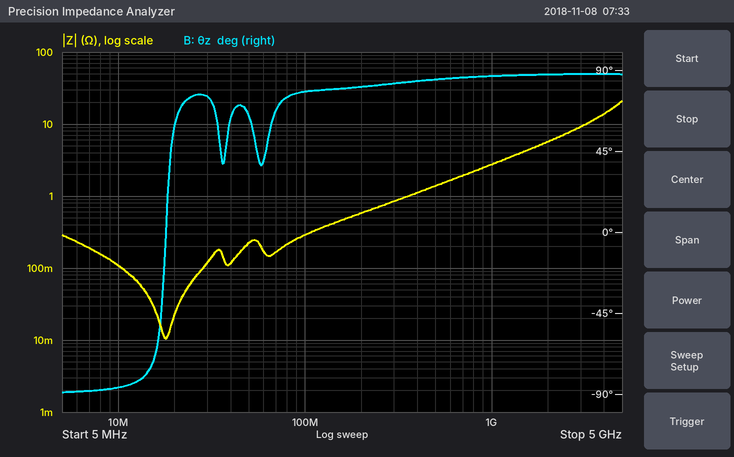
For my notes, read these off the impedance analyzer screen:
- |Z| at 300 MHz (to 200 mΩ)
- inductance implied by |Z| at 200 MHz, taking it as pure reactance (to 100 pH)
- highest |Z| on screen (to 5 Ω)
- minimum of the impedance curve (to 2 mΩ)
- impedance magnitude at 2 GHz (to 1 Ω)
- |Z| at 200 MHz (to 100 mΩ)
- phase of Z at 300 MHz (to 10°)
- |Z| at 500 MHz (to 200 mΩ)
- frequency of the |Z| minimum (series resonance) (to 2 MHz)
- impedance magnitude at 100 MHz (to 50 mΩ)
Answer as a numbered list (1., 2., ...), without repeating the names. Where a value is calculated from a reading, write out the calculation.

1. 800 mΩ
2. L = 600 mΩ/(2π × 200 MHz) ≈ 477 pH, so 500 pH to the nearest 100 pH
3. 20 Ω
4. 10 mΩ
5. 6 Ω
6. 600 mΩ
7. 80°
8. 1.4 Ω
9. 18 MHz
10. 300 mΩ
